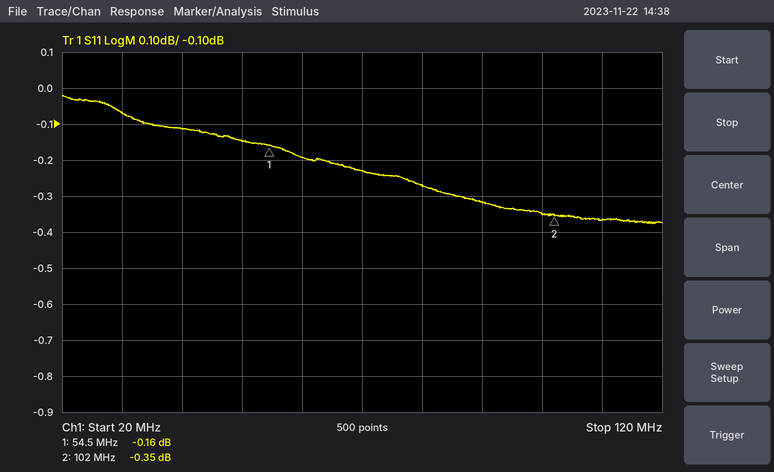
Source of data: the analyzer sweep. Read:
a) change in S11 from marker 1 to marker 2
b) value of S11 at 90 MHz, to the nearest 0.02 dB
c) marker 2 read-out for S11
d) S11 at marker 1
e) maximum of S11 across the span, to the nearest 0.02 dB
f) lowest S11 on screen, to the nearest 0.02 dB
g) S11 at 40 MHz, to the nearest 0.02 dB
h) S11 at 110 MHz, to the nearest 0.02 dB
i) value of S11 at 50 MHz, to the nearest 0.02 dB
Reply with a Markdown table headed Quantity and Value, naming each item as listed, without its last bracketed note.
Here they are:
| Quantity | Value |
|---|---|
| change in S11 from marker 1 to marker 2 | -0.19 dB |
| value of S11 at 90 MHz, to the nearest 0.02 dB | -0.32 dB |
| marker 2 read-out for S11 | -0.35 dB |
| S11 at marker 1 | -0.16 dB |
| maximum of S11 across the span, to the nearest 0.02 dB | -0.02 dB |
| lowest S11 on screen, to the nearest 0.02 dB | -0.38 dB |
| S11 at 40 MHz, to the nearest 0.02 dB | -0.12 dB |
| S11 at 110 MHz, to the nearest 0.02 dB | -0.36 dB |
| value of S11 at 50 MHz, to the nearest 0.02 dB | -0.14 dB |
